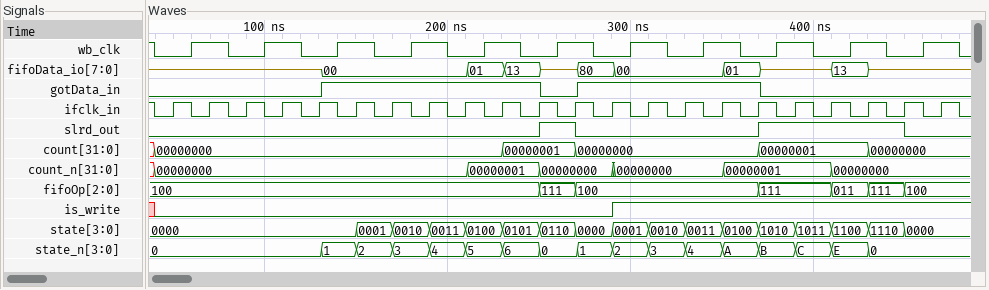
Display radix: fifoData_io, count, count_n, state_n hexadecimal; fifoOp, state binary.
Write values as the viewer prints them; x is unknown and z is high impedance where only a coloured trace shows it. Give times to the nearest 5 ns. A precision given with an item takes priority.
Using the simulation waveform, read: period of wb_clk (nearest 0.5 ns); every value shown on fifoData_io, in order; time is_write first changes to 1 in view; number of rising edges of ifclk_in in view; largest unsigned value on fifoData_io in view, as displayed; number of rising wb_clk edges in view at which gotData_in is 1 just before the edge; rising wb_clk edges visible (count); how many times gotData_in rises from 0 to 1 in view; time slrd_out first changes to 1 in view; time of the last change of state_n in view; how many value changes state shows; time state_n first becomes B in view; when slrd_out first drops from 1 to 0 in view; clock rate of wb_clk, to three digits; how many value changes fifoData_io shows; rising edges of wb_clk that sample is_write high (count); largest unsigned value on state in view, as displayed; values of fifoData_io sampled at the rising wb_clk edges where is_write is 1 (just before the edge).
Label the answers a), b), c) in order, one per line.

a) 40 ns
b) z, 00, 01, 13, z, 80, 00, 01, z, 13, z
c) 290 ns
d) 22
e) 80
f) 5
g) 11
h) 2
i) 250 ns
j) 430 ns
k) 16
l) 370 ns
m) 270 ns
n) 25.0 MHz
o) 10
p) 5
q) 1110
r) 00, 00, z, 13, z
